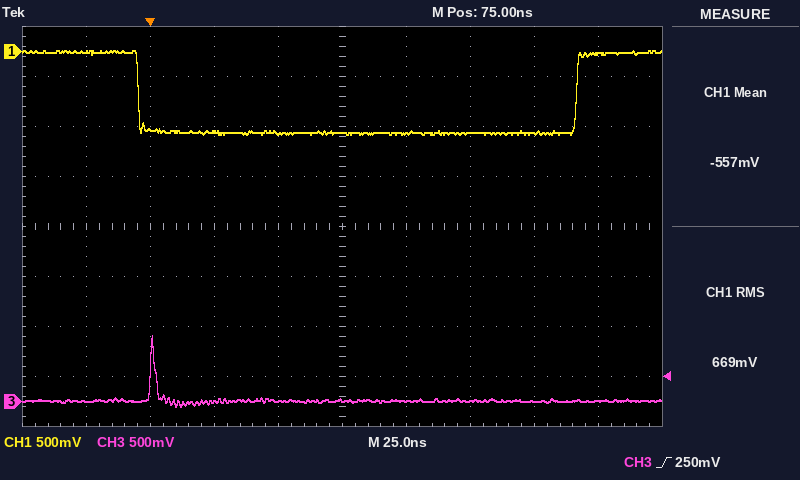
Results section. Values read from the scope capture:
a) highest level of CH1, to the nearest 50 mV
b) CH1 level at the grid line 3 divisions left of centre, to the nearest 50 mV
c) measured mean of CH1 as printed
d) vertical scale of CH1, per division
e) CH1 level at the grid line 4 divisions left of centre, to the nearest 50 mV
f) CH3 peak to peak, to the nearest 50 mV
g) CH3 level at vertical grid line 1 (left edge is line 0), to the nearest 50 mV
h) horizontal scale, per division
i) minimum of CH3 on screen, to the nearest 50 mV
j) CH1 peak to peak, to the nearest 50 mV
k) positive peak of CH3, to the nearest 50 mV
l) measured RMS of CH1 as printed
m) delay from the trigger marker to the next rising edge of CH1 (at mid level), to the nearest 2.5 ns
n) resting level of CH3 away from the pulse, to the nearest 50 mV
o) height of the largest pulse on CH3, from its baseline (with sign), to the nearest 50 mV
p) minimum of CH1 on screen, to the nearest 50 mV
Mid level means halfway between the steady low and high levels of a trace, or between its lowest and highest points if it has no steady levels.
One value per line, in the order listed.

0 mV
-800 mV
-557 mV
500 mV
0 mV
700 mV
0 mV
25 ns
-50 mV
850 mV
650 mV
669 mV
167.5 ns
0 mV
+650 mV
-850 mV
